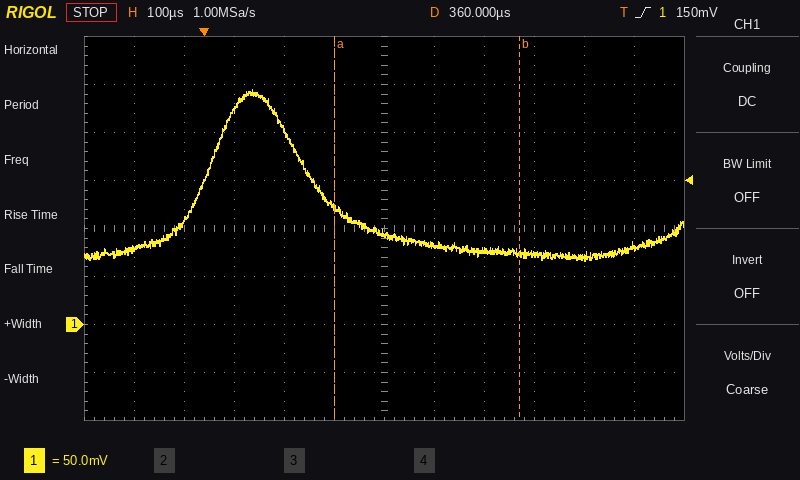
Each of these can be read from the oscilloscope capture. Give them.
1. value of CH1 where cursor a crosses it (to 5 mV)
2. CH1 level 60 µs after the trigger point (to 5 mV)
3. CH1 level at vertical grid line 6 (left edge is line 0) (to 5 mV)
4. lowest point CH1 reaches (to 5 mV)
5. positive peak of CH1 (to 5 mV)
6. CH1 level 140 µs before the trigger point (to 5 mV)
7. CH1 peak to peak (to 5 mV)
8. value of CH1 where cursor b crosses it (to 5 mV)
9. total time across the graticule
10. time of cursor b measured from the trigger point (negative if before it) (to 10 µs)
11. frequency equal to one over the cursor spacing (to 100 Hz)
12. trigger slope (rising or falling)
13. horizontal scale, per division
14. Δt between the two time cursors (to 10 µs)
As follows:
125 mV
225 mV
95 mV
65 mV
245 mV
80 mV
180 mV
75 mV
1.2 ms
+630 µs
2.7 kHz
rising
100 µs
370 µs
